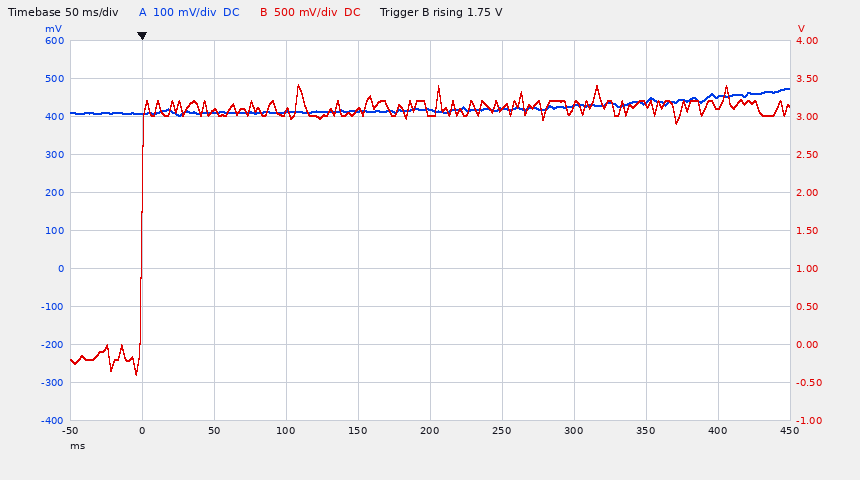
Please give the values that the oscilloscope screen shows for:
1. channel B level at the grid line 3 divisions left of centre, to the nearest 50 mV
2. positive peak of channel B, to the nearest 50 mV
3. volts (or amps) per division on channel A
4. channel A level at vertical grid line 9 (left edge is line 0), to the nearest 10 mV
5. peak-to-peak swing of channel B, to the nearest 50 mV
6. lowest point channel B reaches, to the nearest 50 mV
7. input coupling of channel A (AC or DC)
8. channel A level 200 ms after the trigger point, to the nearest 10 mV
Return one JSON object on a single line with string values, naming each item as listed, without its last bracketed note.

{"channel B level at the grid line 3 divisions left of centre, to the nearest 50 mV": "3.10 V", "positive peak of channel B, to the nearest 50 mV": "3.40 V", "volts (or amps) per division on channel A": "100 mV", "channel A level at vertical grid line 9 (left edge is line 0), to the nearest 10 mV": "450 mV", "peak-to-peak swing of channel B, to the nearest 50 mV": "3.80 V", "lowest point channel B reaches, to the nearest 50 mV": "-400 mV", "input coupling of channel A": "DC", "channel A level 200 ms after the trigger point, to the nearest 10 mV": "420 mV"}
